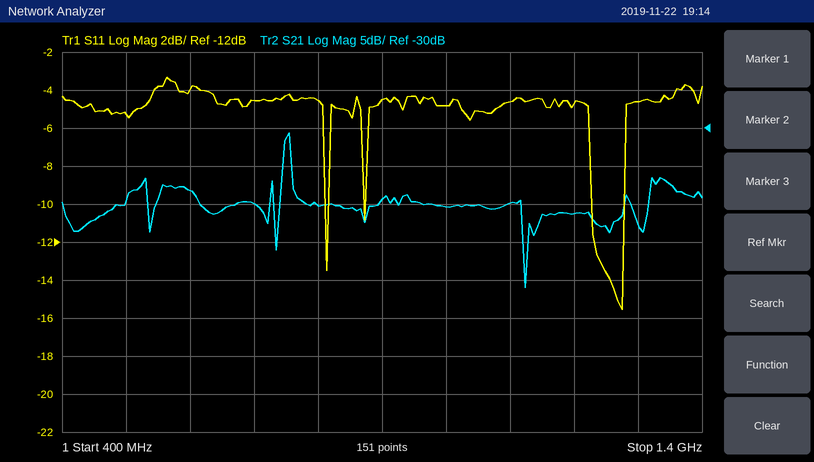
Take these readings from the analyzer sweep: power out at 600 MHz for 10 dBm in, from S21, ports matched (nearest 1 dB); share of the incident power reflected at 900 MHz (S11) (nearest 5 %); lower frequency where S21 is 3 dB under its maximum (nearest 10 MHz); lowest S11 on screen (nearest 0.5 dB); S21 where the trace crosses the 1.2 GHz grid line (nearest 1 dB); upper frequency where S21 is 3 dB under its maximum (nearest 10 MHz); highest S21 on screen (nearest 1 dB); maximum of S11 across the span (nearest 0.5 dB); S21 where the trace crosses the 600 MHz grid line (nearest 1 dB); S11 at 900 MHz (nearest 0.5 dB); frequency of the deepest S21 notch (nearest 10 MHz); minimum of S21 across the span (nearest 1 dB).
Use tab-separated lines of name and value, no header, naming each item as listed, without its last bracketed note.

power out at 600 MHz for 10 dBm in, from S21, ports matched	-28 dBm
share of the incident power reflected at 900 MHz (S11)	35 %
lower frequency where S21 is 3 dB under its maximum	750 MHz
lowest S11 on screen	-15.5 dB
S21 where the trace crosses the 1.2 GHz grid line	-41 dB
upper frequency where S21 is 3 dB under its maximum	760 MHz
highest S21 on screen	-31 dB
maximum of S11 across the span	-3.5 dB
S21 where the trace crosses the 600 MHz grid line	-38 dB
S11 at 900 MHz	-4.5 dB
frequency of the deepest S21 notch	1.12 GHz
minimum of S21 across the span	-51 dB
